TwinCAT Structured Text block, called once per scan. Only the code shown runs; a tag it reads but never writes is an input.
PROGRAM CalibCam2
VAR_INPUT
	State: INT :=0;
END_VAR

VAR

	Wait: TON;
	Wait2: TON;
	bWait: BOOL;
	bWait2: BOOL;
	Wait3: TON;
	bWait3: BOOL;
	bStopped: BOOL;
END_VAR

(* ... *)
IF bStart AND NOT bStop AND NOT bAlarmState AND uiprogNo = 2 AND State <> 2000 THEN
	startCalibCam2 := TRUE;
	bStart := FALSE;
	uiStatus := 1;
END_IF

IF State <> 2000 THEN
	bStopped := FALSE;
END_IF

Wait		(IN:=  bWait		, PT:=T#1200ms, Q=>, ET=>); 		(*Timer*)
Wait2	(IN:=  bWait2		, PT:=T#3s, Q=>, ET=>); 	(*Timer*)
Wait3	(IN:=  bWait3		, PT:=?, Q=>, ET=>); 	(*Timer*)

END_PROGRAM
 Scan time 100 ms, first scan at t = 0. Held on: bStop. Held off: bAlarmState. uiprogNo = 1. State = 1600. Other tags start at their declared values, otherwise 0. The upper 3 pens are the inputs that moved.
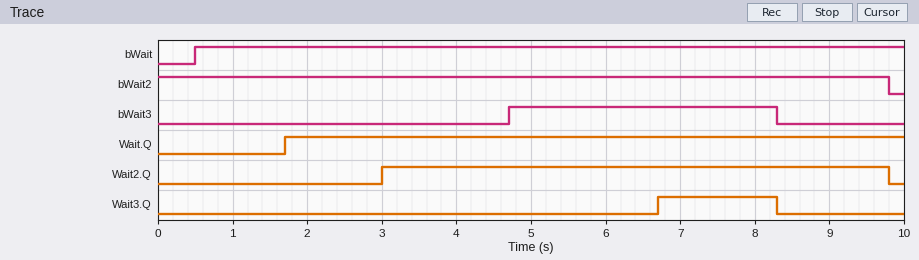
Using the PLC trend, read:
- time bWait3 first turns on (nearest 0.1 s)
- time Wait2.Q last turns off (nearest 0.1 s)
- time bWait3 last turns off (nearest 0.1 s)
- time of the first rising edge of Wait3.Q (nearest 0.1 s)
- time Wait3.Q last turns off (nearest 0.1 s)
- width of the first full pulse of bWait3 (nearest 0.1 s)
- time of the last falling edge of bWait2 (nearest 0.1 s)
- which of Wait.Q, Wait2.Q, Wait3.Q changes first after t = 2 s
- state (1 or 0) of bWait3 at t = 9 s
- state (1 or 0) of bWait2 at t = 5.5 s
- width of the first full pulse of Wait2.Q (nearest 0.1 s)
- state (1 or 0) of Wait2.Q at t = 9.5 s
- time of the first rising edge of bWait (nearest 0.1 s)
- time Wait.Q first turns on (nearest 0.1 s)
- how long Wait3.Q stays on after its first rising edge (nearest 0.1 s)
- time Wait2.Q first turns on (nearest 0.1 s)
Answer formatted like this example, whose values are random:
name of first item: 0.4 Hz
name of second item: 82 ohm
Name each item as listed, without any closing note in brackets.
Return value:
time bWait3 first turns on: 4.7 s
time Wait2.Q last turns off: 9.8 s
time bWait3 last turns off: 8.3 s
time of the first rising edge of Wait3.Q: 6.7 s
time Wait3.Q last turns off: 8.3 s
width of the first full pulse of bWait3: 3.6 s
time of the last falling edge of bWait2: 9.8 s
which of Wait.Q, Wait2.Q, Wait3.Q changes first after t = 2 s: Wait2.Q
state (1 or 0) of bWait3 at t = 9 s: 0
state (1 or 0) of bWait2 at t = 5.5 s: 1
width of the first full pulse of Wait2.Q: 6.8 s
state (1 or 0) of Wait2.Q at t = 9.5 s: 1
time of the first rising edge of bWait: 0.5 s
time Wait.Q first turns on: 1.7 s
how long Wait3.Q stays on after its first rising edge: 1.6 s
time Wait2.Q first turns on: 3.0 s
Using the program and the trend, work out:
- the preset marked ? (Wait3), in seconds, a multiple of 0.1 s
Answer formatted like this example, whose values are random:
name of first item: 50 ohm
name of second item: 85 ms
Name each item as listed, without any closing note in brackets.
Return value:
the preset marked ? (Wait3), in seconds, a multiple of 0.1 s: 2.0 s
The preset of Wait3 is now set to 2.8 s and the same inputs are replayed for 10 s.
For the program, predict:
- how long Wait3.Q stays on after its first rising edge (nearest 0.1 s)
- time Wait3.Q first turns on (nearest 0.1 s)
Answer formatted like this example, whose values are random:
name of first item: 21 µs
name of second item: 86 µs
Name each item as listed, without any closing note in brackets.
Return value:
how long Wait3.Q stays on after its first rising edge: 0.8 s
time Wait3.Q first turns on: 7.5 s
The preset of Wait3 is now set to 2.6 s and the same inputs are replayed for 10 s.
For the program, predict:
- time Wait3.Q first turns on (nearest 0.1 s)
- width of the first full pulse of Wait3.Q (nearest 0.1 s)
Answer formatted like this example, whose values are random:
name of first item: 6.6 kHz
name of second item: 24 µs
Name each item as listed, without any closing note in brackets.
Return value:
time Wait3.Q first turns on: 7.3 s
width of the first full pulse of Wait3.Q: 1.0 s
